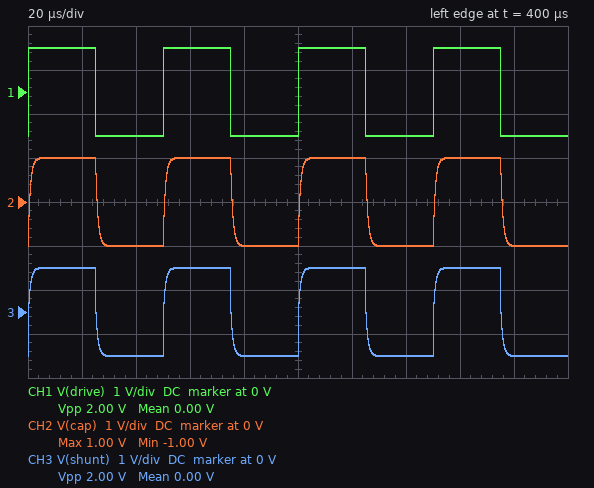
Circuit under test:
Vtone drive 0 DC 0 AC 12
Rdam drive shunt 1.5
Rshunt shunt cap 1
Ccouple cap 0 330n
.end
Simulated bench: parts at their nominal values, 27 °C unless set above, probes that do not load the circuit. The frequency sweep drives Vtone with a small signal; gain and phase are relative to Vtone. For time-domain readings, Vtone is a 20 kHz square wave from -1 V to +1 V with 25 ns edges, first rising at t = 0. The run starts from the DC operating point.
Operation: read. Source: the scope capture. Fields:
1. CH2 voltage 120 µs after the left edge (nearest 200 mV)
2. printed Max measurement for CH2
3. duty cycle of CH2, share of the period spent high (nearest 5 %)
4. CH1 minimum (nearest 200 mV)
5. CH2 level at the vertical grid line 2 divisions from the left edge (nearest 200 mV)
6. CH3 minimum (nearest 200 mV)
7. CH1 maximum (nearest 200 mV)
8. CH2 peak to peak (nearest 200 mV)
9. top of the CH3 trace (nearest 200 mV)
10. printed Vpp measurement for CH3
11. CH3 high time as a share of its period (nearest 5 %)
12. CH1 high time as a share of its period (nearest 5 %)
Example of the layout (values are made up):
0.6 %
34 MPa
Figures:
1.0 V
1.00 V
50 %
-1.0 V
-1.0 V
-1.0 V
1.0 V
2.0 V
1.0 V
2.00 V
50 %
50 %
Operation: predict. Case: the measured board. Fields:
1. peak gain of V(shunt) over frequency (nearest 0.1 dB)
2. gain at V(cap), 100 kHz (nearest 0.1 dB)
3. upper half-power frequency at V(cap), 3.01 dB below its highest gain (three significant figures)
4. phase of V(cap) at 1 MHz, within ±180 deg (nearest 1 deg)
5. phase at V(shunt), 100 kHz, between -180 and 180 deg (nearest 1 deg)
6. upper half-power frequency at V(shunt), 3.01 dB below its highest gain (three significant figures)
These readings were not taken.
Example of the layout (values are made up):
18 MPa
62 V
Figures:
0 dB
-1.0 dB
193 kHz
-79 deg
-16 deg
234 kHz
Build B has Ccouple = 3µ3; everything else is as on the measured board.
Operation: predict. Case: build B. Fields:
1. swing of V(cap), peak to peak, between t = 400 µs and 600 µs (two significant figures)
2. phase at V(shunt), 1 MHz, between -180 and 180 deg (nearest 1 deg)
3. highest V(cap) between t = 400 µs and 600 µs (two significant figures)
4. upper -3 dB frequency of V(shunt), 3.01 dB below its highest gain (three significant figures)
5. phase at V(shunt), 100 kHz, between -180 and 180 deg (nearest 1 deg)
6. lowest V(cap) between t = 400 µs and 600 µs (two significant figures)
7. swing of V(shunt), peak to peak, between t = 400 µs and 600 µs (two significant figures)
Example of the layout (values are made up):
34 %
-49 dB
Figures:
1.8 V
-2 deg
910 mV
23.4 kHz
-15 deg
-910 mV
1.9 V
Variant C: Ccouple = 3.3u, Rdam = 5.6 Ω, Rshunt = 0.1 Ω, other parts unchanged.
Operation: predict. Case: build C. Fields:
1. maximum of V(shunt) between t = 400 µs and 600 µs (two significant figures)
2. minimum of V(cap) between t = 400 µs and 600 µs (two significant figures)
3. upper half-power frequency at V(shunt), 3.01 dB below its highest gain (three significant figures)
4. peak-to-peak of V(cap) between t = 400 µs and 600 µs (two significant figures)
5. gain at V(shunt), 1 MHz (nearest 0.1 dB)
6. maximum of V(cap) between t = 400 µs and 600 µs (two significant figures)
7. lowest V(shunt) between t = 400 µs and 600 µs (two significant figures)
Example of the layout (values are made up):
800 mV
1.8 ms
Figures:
590 mV
-580 mV
8.46 kHz
1.2 V
-34.2 dB
580 mV
-590 mV
